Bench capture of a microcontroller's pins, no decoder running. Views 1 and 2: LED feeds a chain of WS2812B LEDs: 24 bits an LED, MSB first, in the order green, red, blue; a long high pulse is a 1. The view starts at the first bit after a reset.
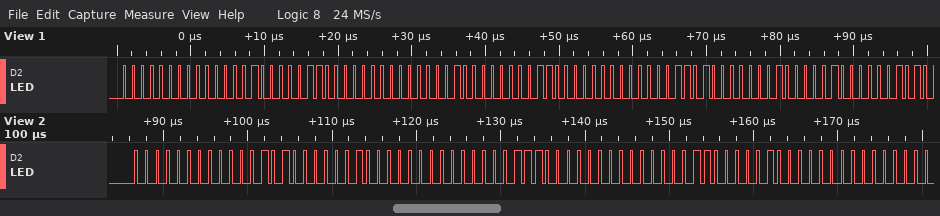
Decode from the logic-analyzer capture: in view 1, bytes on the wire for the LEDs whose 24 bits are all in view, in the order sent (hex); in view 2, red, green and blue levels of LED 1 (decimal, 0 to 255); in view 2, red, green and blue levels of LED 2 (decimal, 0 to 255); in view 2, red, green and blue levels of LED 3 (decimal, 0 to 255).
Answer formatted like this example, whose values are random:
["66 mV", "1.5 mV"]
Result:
["00 02 0C 00 08 06 00 0D 01", "10, 0, 4", "14, 0, 0", "8, 6, 0"]
